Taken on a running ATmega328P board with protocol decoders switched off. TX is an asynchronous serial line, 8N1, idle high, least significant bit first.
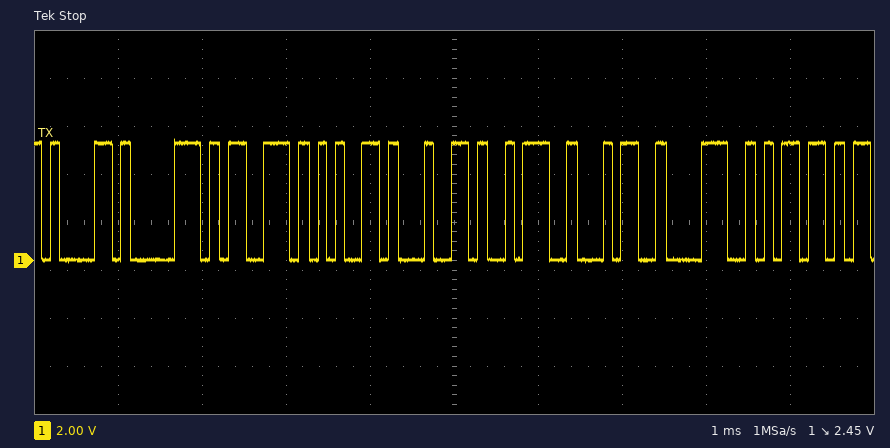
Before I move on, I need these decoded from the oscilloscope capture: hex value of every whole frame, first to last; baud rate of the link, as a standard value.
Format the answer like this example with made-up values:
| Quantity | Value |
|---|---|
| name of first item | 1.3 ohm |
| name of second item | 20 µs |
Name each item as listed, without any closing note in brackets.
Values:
| Quantity | Value |
|---|---|
| hex value of every whole frame, first to last | 0x61 0x70 0x73 0x65 0x64 0x3A 0x34 0x38 0x6D |
| baud rate of the link, as a standard value | 9600 baud |
